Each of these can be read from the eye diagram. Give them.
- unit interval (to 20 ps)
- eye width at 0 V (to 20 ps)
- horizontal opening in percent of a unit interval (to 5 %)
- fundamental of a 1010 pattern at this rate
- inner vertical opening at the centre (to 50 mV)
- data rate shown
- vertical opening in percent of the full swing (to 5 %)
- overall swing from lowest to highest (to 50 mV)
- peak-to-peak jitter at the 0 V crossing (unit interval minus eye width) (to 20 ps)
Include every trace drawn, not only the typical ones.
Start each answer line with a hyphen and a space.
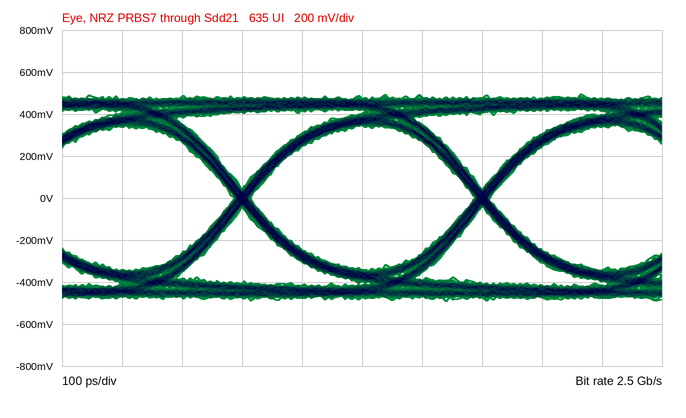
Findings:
- 400 ps
- 380 ps
- 95 %
- 1.25 GHz
- 700 mV
- 2.5 Gb/s
- 70 %
- 1.00 V
- 20 ps
